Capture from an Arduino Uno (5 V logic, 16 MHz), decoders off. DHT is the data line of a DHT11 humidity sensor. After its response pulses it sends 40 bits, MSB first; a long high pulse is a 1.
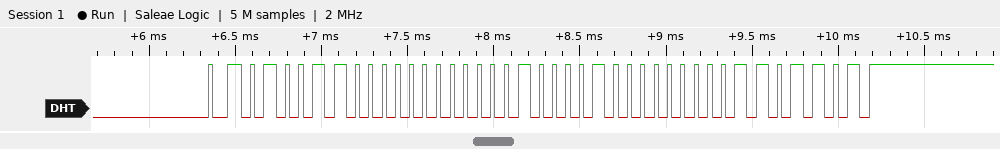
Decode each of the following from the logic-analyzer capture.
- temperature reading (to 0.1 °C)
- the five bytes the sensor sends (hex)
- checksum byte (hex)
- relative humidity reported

33.0 °C
4C 00 21 00 6D
0x6D
76 %
